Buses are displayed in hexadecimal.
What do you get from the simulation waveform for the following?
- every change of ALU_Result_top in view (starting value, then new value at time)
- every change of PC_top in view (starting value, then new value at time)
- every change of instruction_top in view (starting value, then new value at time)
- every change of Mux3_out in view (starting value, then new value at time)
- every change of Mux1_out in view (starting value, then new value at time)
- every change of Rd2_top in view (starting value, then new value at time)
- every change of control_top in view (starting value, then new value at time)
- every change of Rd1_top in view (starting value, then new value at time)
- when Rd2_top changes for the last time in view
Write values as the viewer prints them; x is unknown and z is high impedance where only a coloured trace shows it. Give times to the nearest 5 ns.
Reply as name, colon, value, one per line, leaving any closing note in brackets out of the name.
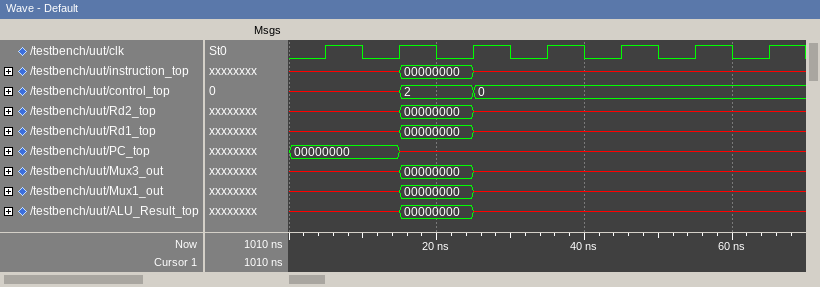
every change of ALU_Result_top in view: x, 00000000 at 15 ns, x at 25 ns
every change of PC_top in view: 00000000, x at 15 ns
every change of instruction_top in view: x, 00000000 at 15 ns, x at 25 ns
every change of Mux3_out in view: x, 00000000 at 15 ns, x at 25 ns
every change of Mux1_out in view: x, 00000000 at 15 ns, x at 25 ns
every change of Rd2_top in view: x, 00000000 at 15 ns, x at 25 ns
every change of control_top in view: x, 2 at 15 ns, 0 at 25 ns
every change of Rd1_top in view: x, 00000000 at 15 ns, x at 25 ns
when Rd2_top changes for the last time in view: 25 ns
